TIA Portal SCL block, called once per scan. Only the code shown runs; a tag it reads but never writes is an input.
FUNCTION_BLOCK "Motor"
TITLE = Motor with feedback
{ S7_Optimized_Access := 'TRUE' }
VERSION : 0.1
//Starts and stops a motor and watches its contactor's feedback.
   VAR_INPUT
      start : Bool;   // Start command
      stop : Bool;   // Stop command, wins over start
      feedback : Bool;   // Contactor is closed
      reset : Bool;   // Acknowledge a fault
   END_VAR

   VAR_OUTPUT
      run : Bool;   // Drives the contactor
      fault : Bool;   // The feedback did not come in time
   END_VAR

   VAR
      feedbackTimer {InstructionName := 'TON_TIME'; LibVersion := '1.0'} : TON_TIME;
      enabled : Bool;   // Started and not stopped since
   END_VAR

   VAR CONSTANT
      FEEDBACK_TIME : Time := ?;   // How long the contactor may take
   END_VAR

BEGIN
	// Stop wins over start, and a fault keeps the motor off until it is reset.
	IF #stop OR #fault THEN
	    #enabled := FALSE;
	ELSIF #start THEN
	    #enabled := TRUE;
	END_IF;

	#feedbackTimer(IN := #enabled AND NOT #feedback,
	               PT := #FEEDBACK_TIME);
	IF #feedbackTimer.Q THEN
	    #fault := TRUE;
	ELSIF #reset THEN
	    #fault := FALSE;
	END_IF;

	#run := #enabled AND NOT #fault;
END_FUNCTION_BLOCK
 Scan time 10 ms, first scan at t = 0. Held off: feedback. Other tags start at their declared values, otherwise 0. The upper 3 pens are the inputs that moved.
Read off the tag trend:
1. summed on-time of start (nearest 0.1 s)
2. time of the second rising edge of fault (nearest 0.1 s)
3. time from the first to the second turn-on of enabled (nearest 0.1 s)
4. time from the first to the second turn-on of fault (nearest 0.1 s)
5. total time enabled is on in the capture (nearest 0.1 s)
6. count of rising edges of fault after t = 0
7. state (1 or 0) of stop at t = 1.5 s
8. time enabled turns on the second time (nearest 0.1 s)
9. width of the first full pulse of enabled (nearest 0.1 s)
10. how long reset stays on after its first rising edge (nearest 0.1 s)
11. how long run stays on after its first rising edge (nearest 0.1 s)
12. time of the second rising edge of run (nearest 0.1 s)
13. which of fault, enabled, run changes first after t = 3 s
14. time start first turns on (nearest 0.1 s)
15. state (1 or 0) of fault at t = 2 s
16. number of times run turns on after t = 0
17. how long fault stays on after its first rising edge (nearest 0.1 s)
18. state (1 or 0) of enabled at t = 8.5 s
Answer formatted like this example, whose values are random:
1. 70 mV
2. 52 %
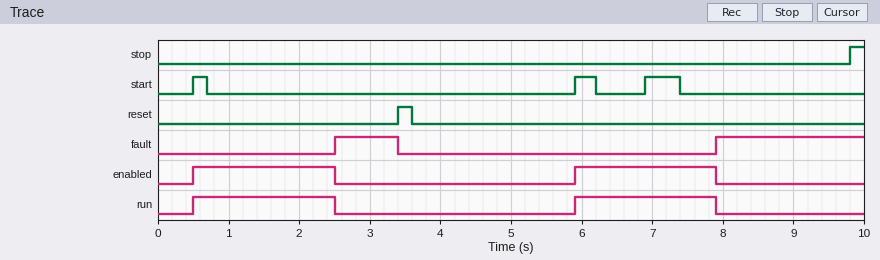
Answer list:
1. 1.0 s
2. 7.9 s
3. 5.4 s
4. 5.4 s
5. 4.0 s
6. 2
7. 0
8. 5.9 s
9. 2.0 s
10. 0.2 s
11. 2.0 s
12. 5.9 s
13. fault
14. 0.5 s
15. 0
16. 2
17. 0.9 s
18. 0
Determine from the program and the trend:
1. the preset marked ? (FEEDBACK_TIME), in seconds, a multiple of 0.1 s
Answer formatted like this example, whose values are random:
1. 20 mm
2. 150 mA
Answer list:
1. 2.0 s
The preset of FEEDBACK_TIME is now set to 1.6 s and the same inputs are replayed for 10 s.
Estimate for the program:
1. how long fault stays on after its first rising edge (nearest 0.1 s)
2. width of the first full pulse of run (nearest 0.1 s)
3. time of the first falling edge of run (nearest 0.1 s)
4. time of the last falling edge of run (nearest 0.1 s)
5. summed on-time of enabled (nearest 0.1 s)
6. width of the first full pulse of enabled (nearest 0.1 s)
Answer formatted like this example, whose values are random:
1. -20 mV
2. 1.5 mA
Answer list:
1. 1.3 s
2. 1.6 s
3. 2.1 s
4. 7.5 s
5. 3.2 s
6. 1.6 s
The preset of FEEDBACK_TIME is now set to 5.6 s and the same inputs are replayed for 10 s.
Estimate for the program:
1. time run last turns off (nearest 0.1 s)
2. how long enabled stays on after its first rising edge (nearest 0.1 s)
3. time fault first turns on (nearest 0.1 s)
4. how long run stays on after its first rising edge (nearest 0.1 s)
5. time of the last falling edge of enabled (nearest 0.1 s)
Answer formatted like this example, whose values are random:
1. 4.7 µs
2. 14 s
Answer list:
1. 6.1 s
2. 5.6 s
3. 6.1 s
4. 5.6 s
5. 6.1 s
